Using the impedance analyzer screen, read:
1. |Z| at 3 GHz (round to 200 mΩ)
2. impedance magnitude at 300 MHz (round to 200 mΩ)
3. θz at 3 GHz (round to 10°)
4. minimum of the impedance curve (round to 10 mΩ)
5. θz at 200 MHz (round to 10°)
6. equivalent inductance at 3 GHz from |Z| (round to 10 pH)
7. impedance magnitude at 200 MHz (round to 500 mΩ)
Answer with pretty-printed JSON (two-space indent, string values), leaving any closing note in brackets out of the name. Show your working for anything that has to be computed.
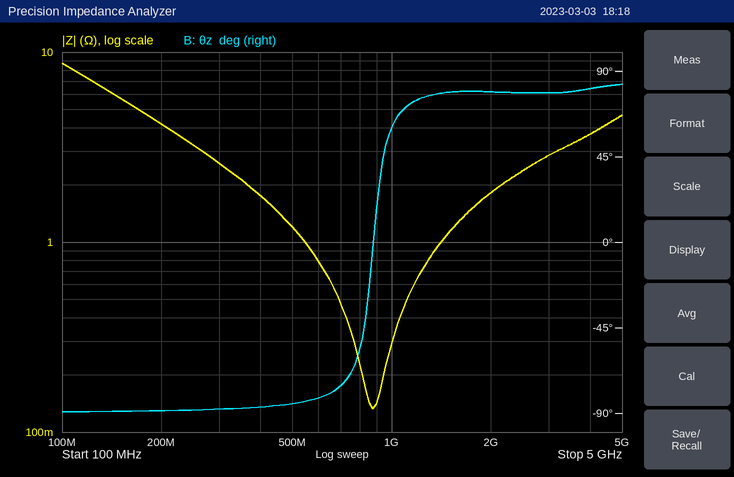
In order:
{
  "|Z| at 3 GHz": "2.8 Ω",
  "impedance magnitude at 300 MHz": "2.6 Ω",
  "θz at 3 GHz": "80°",
  "minimum of the impedance curve": "130 mΩ",
  "θz at 200 MHz": "-90°",
  "equivalent inductance at 3 GHz from |Z|": "L = 2.8 Ω/(2π × 3 GHz) ≈ 149 pH, so 150 pH to the nearest 10 pH",
  "impedance magnitude at 200 MHz": "4.0 Ω"
}
